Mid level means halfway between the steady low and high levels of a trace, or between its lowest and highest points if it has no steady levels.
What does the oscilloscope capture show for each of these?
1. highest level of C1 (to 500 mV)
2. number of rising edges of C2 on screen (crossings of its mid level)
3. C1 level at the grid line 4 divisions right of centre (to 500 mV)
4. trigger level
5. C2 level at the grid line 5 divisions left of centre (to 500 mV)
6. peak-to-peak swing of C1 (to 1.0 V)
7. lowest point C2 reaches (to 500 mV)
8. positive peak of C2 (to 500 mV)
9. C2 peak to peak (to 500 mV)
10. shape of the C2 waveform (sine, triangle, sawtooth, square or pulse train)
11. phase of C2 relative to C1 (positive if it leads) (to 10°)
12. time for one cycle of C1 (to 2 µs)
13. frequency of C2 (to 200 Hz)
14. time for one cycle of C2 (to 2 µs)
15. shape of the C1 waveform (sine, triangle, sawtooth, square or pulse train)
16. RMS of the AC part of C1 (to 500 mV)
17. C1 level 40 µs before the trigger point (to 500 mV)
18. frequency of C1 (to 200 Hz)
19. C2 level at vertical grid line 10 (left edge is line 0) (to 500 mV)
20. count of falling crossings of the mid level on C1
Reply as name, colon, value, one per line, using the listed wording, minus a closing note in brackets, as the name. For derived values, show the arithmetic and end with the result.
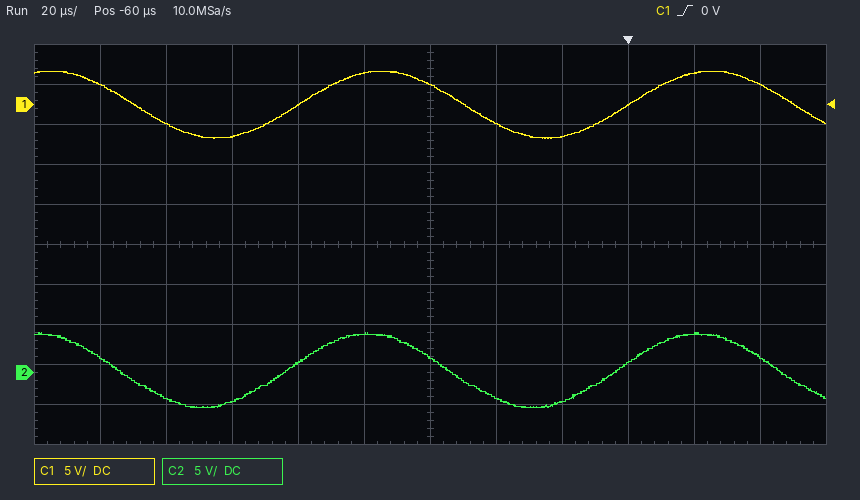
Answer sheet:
highest level of C1: 4.0 V
number of rising edges of C2 on screen: 2
C1 level at the grid line 4 divisions right of centre: 4.0 V
trigger level: 0 V
C2 level at the grid line 5 divisions left of centre: 2.0 V
peak-to-peak swing of C1: 8.0 V
lowest point C2 reaches: -4.5 V
positive peak of C2: 5.0 V
C2 peak to peak: 5.0 V − (-4.5 V) = 9.5 V
shape of the C2 waveform: sine
phase of C2 relative to C1 (positive if it leads): +10°
time for one cycle of C1: 100 µs
frequency of C2: 1 / 100 µs ≈ 10.0 kHz
time for one cycle of C2: 100 µs
shape of the C1 waveform: sine
RMS of the AC part of C1: 8.0 V / (2√2) ≈ 2.83 V, so 3.0 V to the nearest 500 mV
C1 level 40 µs before the trigger point: -2.5 V
frequency of C1: 1 / 100 µs ≈ 10.0 kHz
C2 level at vertical grid line 10 (left edge is line 0): 5.0 V
count of falling crossings of the mid level on C1: 3
